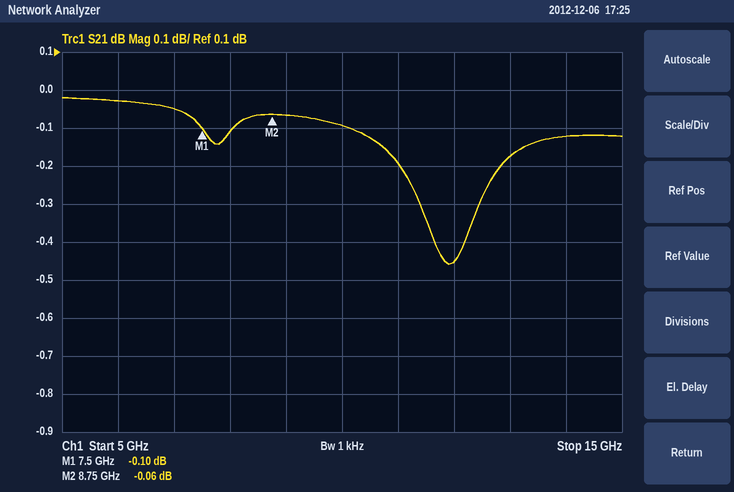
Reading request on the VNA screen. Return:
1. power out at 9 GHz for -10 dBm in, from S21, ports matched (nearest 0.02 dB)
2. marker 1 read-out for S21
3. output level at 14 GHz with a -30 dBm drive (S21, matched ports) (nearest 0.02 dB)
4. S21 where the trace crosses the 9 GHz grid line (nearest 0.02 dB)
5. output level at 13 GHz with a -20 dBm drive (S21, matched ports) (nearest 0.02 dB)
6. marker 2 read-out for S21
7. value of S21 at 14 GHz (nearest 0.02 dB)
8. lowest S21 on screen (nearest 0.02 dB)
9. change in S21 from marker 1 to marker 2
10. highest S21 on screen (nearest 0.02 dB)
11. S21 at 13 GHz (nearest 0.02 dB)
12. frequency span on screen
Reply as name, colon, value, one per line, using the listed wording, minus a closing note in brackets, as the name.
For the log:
power out at 9 GHz for -10 dBm in, from S21, ports matched: -10.06 dBm
marker 1 read-out for S21: -0.10 dB
output level at 14 GHz with a -30 dBm drive (S21, matched ports): -30.12 dBm
S21 where the trace crosses the 9 GHz grid line: -0.06 dB
output level at 13 GHz with a -20 dBm drive (S21, matched ports): -20.18 dBm
marker 2 read-out for S21: -0.06 dB
value of S21 at 14 GHz: -0.12 dB
lowest S21 on screen: -0.46 dB
change in S21 from marker 1 to marker 2: 0.04 dB
highest S21 on screen: -0.02 dB
S21 at 13 GHz: -0.18 dB
frequency span on screen: 10 GHz
